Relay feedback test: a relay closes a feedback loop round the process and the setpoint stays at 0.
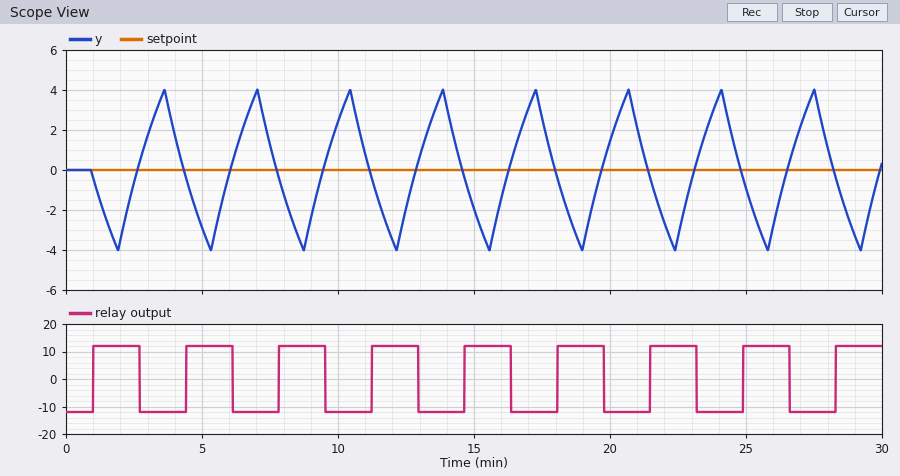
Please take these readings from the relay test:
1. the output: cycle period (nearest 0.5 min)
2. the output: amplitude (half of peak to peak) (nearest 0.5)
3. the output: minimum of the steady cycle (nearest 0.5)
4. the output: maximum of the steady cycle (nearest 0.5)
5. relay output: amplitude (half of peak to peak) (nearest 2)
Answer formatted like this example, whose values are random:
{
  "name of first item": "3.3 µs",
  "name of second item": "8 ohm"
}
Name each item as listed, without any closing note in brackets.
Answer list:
{
  "the output: cycle period": "3.5 min",
  "the output: amplitude (half of peak to peak)": "4.0",
  "the output: minimum of the steady cycle": "-4.0",
  "the output: maximum of the steady cycle": "4.0",
  "relay output: amplitude (half of peak to peak)": "12"
}
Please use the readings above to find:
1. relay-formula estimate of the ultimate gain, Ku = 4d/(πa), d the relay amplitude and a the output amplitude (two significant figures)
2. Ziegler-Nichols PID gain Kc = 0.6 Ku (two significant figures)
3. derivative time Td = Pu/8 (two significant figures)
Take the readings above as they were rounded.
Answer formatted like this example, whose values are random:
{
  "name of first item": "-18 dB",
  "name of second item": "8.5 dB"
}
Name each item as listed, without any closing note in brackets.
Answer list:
{
  "relay-formula estimate of the ultimate gain, Ku = 4d/(πa), d the relay amplitude and a the output amplitude": "3.8",
  "Ziegler-Nichols PID gain Kc = 0.6 Ku": "2.3",
  "derivative time Td = Pu/8": "0.44 min"
}
